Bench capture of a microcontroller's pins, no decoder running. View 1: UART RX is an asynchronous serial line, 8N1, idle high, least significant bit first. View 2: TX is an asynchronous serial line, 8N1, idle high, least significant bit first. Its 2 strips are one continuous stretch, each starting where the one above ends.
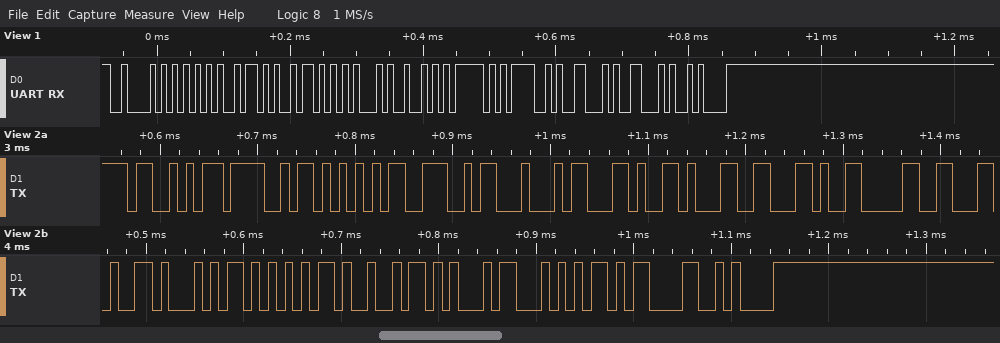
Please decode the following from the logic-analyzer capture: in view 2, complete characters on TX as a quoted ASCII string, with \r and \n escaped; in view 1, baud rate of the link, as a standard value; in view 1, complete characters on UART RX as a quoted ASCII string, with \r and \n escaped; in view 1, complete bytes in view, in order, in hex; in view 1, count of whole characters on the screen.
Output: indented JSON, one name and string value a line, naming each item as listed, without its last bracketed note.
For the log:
{
  "in view 2, complete characters on TX as a quoted ASCII string, with \\r and \\n escaped": "\"SOUND,1,0,QUIET\\r\\n\"",
  "in view 1, baud rate of the link, as a standard value": "115200 baud",
  "in view 1, complete characters on UART RX as a quoted ASCII string, with \\r and \\n escaped": "\"BUZZER_OFF\\n\"",
  "in view 1, complete bytes in view, in order, in hex": "0x42 0x55 0x5A 0x5A 0x45 0x52 0x5F 0x4F 0x46 0x46 0x0A",
  "in view 1, count of whole characters on the screen": "11"
}
